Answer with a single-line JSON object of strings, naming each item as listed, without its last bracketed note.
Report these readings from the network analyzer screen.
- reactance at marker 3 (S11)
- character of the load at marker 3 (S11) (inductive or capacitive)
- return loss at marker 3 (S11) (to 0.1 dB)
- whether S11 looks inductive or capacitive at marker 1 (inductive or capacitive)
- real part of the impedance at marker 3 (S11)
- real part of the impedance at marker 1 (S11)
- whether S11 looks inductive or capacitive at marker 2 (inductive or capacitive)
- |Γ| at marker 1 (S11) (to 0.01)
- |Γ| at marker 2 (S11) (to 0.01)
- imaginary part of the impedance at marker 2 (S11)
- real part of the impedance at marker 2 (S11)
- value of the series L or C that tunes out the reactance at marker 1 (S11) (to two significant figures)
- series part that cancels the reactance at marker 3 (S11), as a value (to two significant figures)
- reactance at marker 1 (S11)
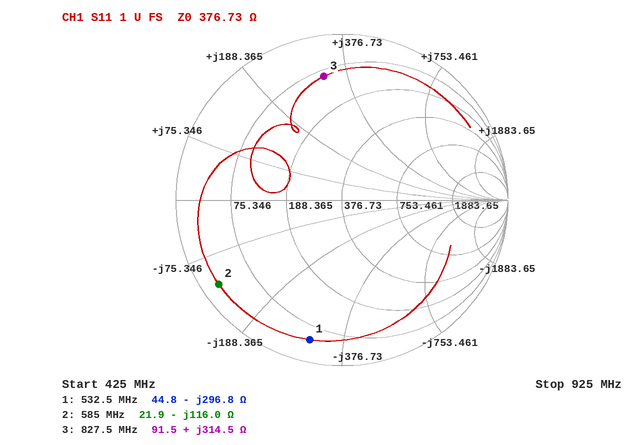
{"reactance at marker 3": "+314.5 Ω", "character of the load at marker 3 (S11)": "inductive", "return loss at marker 3 (S11)": "2.5 dB", "whether S11 looks inductive or capacitive at marker 1": "capacitive", "real part of the impedance at marker 3": "91.5 Ω", "real part of the impedance at marker 1": "44.8 Ω", "whether S11 looks inductive or capacitive at marker 2": "capacitive", "|Γ| at marker 1 (S11)": "0.86", "|Γ| at marker 2 (S11)": "0.90", "imaginary part of the impedance at marker 2": "-116.0 Ω", "real part of the impedance at marker 2": "21.9 Ω", "value of the series L or C that tunes out the reactance at marker 1 (S11)": "89 nH", "series part that cancels the reactance at marker 3 (S11), as a value": "610 fF", "reactance at marker 1": "-296.8 Ω"}
